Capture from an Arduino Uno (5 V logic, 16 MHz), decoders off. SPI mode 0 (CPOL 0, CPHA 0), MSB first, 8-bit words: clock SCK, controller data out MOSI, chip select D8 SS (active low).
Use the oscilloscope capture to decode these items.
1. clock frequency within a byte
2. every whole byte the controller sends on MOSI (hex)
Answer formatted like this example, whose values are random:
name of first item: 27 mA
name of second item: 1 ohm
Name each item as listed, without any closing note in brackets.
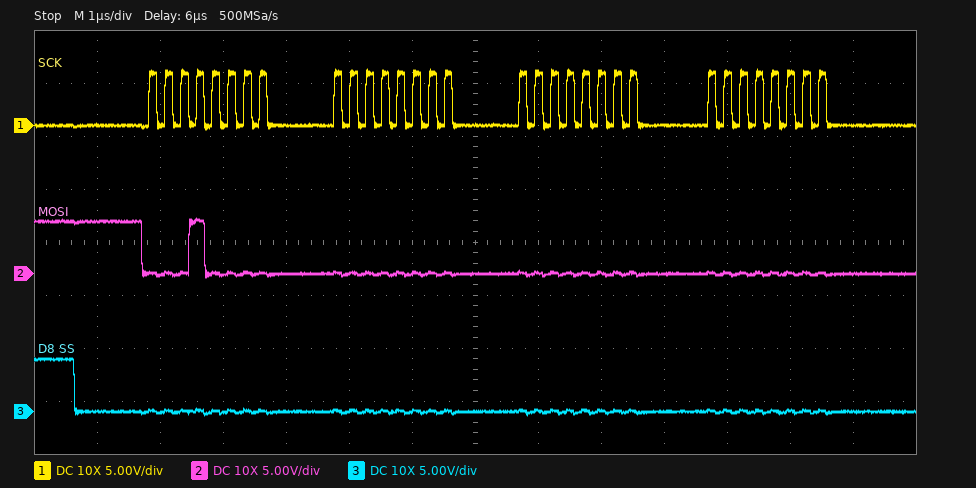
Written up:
clock frequency within a byte: 4 MHz
every whole byte the controller sends on MOSI: 10 00 00 00
